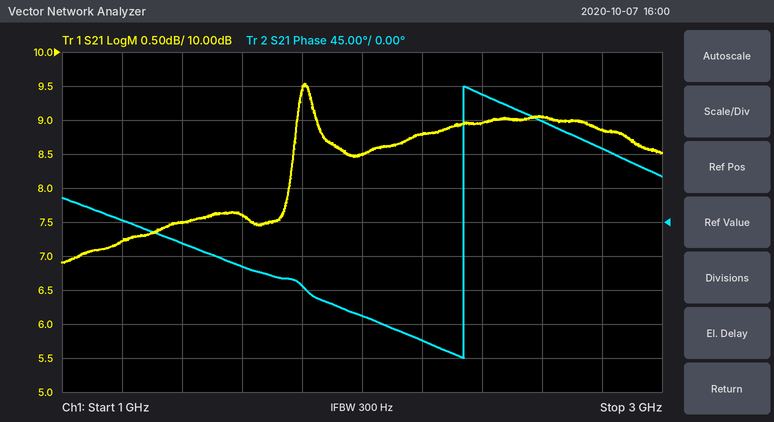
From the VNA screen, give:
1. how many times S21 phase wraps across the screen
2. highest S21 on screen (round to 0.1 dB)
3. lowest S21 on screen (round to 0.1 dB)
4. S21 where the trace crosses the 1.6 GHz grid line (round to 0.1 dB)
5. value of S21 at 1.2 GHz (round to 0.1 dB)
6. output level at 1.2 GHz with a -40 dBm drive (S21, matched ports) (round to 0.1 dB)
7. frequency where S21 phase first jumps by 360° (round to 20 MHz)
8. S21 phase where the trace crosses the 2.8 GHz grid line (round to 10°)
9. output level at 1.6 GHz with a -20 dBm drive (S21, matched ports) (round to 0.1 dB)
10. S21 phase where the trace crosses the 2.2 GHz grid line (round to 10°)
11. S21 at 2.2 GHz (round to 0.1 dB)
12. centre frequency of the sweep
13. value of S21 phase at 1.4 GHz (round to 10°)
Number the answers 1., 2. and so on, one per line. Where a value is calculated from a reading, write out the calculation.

1. 1
2. 9.5 dB
3. 6.9 dB
4. 7.6 dB
5. 7.2 dB
6. -40 dBm + (7.2 dB) = -32.8 dBm
7. 2.34 GHz
8. 100°
9. -20 dBm + (7.6 dB) = -12.4 dBm
10. -160°
11. 8.8 dB
12. 2 GHz
13. -30°
